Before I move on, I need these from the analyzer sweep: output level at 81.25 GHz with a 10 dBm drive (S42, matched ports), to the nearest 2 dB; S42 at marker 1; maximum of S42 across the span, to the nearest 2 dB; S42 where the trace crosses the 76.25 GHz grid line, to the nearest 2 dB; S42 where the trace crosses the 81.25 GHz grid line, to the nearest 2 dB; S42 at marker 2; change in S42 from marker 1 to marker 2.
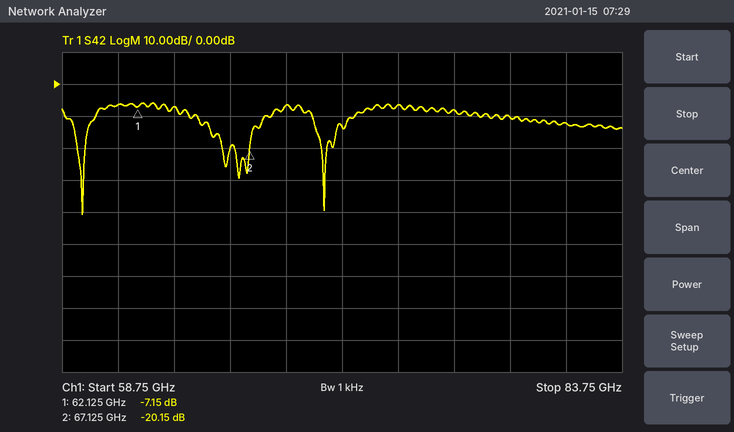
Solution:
-2 dBm
-7.15 dB
-6 dB
-8 dB
-12 dB
-20.15 dB
-13.00 dB
